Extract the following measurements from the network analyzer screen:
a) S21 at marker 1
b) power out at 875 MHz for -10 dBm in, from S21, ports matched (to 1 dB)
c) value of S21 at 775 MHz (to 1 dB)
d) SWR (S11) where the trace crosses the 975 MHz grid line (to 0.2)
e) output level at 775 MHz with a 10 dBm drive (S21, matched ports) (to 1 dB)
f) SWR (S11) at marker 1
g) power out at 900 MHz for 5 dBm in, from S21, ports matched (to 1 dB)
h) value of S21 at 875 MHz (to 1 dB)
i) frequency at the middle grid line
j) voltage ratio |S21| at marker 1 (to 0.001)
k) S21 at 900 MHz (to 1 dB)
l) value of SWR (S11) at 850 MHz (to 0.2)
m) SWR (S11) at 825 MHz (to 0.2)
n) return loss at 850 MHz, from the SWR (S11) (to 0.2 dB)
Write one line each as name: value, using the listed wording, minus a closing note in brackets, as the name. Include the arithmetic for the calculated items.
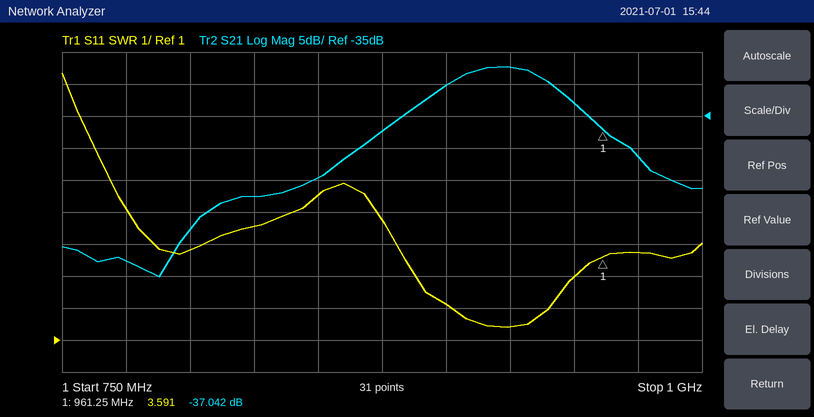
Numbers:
S21 at marker 1: -37.042 dB
power out at 875 MHz for -10 dBm in, from S21, ports matched: -10 dBm + (-37 dB) = -47 dBm
value of S21 at 775 MHz: -58 dB
SWR (S11) where the trace crosses the 975 MHz grid line: 3.8
output level at 775 MHz with a 10 dBm drive (S21, matched ports): 10 dBm + (-58 dB) = -48 dBm
SWR (S11) at marker 1: 3.591
power out at 900 MHz for 5 dBm in, from S21, ports matched: 5 dBm + (-30 dB) = -25 dBm
value of S21 at 875 MHz: -37 dB
frequency at the middle grid line: 875 MHz
voltage ratio |S21| at marker 1: 10^(-37.042/20) ≈ 0.014
S21 at 900 MHz: -30 dB
value of SWR (S11) at 850 MHz: 5.6
SWR (S11) at 825 MHz: 4.6
return loss at 850 MHz, from the SWR (S11): −20 log10((5.6 − 1)/(5.6 + 1)) ≈ 3.14 dB, so 3.2 dB to the nearest 0.2 dB
